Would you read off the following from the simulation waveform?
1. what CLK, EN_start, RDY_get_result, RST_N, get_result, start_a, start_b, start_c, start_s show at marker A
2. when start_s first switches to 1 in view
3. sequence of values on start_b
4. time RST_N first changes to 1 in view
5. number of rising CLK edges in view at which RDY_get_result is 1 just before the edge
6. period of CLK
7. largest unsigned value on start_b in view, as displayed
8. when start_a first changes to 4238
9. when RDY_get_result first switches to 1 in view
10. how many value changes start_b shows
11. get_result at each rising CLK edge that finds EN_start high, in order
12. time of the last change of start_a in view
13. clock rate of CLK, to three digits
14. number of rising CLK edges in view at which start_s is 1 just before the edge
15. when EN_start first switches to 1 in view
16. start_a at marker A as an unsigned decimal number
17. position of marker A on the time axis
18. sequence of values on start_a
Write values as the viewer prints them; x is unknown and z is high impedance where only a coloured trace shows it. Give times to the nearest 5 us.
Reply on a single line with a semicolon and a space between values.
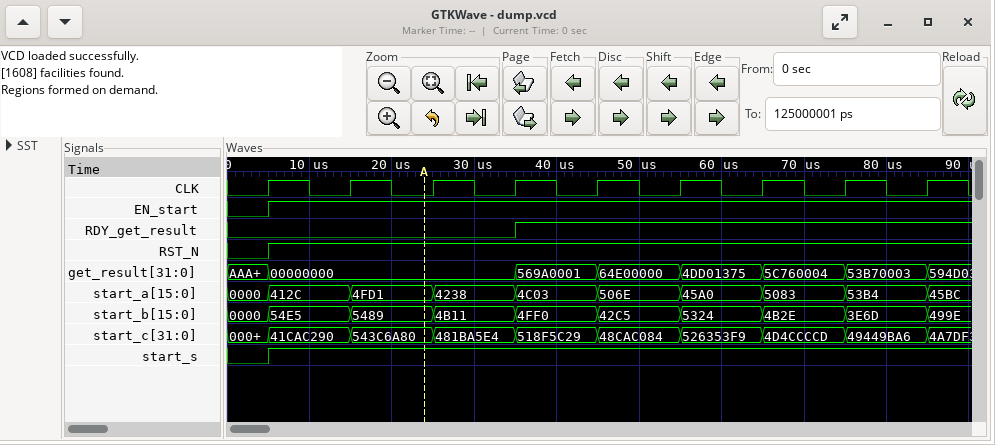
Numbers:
CLK=0, EN_start=1, RDY_get_result=0, RST_N=1, get_result=00000000, start_a=4FD1, start_b=5489, start_c=543C6A80, start_s=1; 5 us; 0000, 54E5, 5489, 4B11, 4FF0, 42C5, 5324, 4B2E, 3E6D, 499E; 5 us; 5; 10 us; 54E5; 25 us; 35 us; 9; 00000000, 00000000, 00000000, 569A0001, 64E00000, 4DD01375, 5C760004, 53B70003; 85 us; 100 kHz; 8; 5 us; 20433; 25 us; 0000, 412C, 4FD1, 4238, 4C03, 506E, 45A0, 5083, 53B4, 45BC
